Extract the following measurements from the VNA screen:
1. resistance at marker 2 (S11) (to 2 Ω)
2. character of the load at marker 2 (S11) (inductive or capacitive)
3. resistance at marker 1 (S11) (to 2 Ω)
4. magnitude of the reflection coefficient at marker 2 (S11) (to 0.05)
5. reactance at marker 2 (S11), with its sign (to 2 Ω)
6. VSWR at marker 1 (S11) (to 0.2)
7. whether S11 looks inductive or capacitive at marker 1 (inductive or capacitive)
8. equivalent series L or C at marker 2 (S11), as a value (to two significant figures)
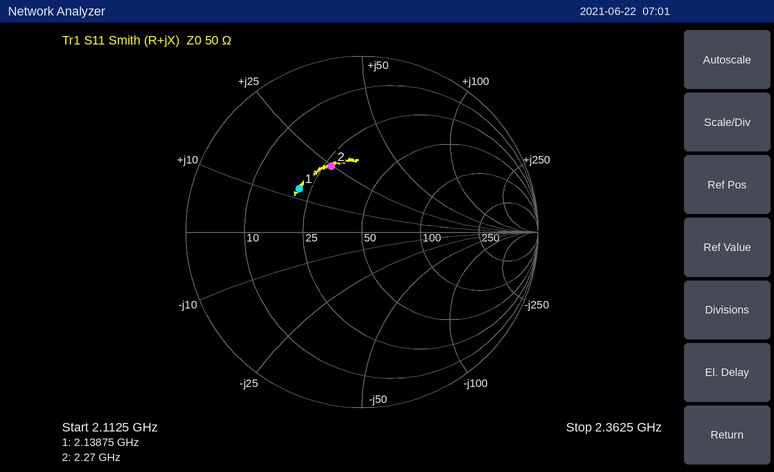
28 Ω
inductive
22 Ω
0.40
+24 Ω
2.6
inductive
1.7 nH
